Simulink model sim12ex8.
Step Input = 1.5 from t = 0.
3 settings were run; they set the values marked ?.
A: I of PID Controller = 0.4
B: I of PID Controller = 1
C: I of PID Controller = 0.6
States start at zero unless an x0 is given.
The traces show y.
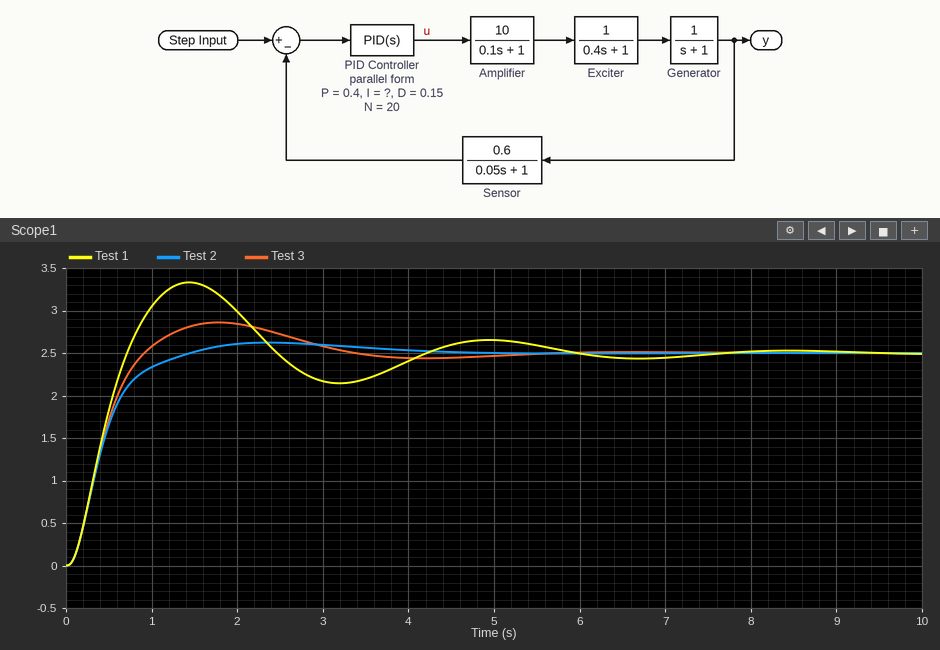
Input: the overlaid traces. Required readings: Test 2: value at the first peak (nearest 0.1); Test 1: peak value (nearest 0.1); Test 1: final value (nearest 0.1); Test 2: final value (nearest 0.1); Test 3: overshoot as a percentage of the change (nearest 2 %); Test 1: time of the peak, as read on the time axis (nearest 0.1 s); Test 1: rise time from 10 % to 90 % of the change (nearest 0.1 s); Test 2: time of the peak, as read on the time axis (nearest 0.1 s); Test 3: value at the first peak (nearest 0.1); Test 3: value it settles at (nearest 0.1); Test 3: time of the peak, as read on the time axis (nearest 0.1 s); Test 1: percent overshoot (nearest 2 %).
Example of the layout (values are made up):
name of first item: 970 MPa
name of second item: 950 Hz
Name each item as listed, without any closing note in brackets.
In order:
Test 2: value at the first peak: 2.6
Test 1: peak value: 3.3
Test 1: final value: 2.5
Test 2: final value: 2.5
Test 3: overshoot as a percentage of the change: 14 %
Test 1: time of the peak, as read on the time axis: 1.4 s
Test 1: rise time from 10 % to 90 % of the change: 0.5 s
Test 2: time of the peak, as read on the time axis: 2.4 s
Test 3: value at the first peak: 2.9
Test 3: value it settles at: 2.5
Test 3: time of the peak, as read on the time axis: 1.8 s
Test 1: percent overshoot: 34 %
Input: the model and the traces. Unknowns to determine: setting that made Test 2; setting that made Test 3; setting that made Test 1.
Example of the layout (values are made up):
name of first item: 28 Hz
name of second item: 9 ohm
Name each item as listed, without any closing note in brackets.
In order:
setting that made Test 2: A
setting that made Test 3: C
setting that made Test 1: B
